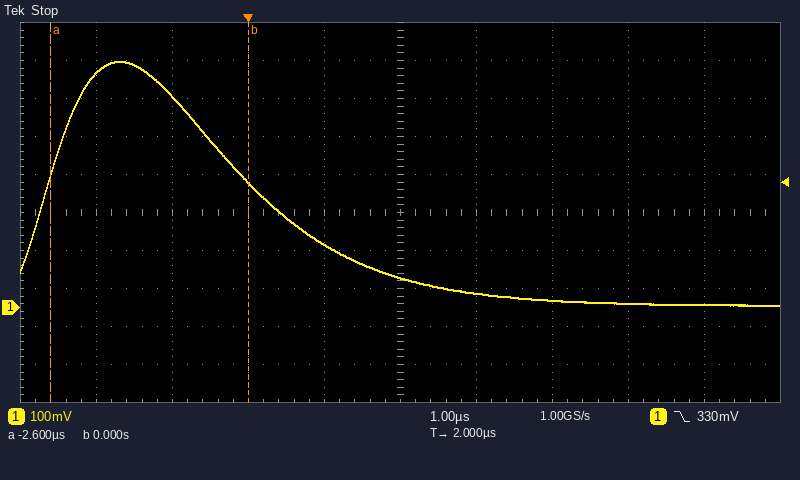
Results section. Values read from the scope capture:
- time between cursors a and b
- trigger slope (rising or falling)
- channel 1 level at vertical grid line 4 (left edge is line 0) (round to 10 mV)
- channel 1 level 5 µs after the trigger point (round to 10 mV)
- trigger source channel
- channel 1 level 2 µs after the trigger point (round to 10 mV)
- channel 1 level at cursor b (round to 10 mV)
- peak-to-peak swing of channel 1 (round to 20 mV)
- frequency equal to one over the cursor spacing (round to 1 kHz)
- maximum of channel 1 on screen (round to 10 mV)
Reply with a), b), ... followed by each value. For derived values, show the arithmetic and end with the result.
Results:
a) 0 s − (-2.6 µs) = 2.6 µs
b) falling
c) 170 mV
d) 10 mV
e) channel 1
f) 80 mV
g) 330 mV
h) 640 mV
i) 1 / 2.6 µs ≈ 385 kHz
j) 650 mV
